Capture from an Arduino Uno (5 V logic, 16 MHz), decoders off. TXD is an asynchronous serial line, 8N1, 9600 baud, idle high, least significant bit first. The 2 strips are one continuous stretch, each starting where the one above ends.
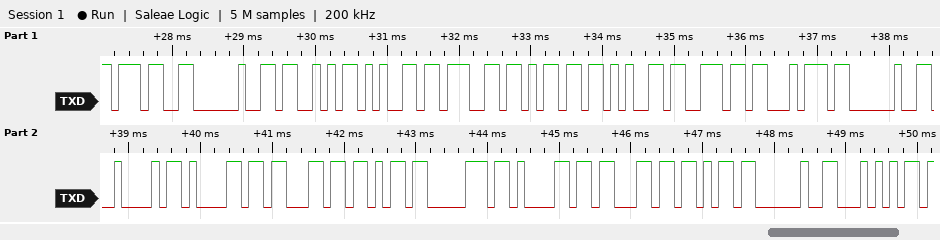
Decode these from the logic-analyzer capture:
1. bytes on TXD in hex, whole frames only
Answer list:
37 20 53 65 67 6D 65 6E 74 20 42 61 63 6B 70 61 63 6B 20 54
